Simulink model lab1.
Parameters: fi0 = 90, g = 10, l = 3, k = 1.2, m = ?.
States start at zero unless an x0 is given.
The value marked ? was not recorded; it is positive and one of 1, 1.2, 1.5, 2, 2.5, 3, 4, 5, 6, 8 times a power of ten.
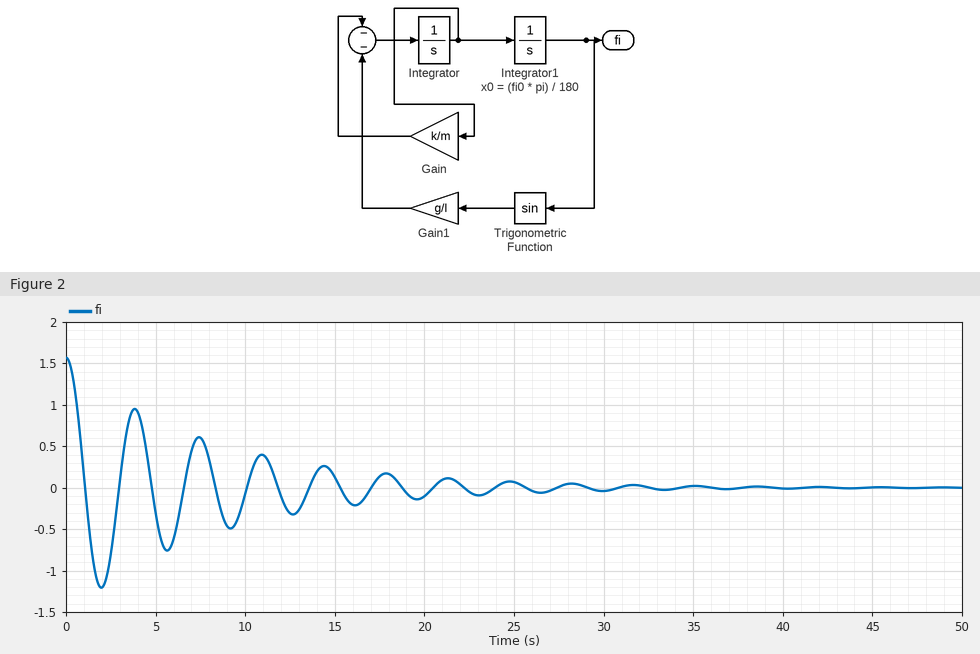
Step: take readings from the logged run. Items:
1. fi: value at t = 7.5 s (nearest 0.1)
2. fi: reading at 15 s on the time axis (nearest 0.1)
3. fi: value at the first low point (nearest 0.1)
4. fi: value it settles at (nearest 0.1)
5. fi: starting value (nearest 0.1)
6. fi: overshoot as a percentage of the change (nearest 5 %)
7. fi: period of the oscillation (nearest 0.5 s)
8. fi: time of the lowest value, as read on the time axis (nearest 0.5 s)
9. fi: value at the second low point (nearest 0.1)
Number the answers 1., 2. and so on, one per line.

1. 0.6
2. 0.1
3. -1.2
4. 0.0
5. 1.6
6. 75 %
7. 3.5 s
8. 2.0 s
9. -0.8
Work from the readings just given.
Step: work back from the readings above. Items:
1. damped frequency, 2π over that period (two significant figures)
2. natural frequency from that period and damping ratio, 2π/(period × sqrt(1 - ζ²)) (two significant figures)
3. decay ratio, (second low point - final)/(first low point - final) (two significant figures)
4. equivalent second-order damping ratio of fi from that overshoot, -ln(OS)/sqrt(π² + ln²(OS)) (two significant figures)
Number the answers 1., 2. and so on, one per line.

1. 1.8 rad/s
2. 1.8 rad/s
3. 0.67
4. 0.091
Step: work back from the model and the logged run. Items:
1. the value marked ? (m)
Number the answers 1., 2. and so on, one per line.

1. 5
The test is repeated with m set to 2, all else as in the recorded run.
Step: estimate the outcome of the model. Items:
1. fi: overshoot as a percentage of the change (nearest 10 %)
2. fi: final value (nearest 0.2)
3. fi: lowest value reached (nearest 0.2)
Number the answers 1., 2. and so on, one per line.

1. 50 %
2. 0.0
3. -0.8
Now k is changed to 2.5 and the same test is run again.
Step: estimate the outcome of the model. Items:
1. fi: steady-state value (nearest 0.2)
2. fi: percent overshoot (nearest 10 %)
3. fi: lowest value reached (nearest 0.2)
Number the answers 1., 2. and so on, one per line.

1. 0.0
2. 60 %
3. -1.0
